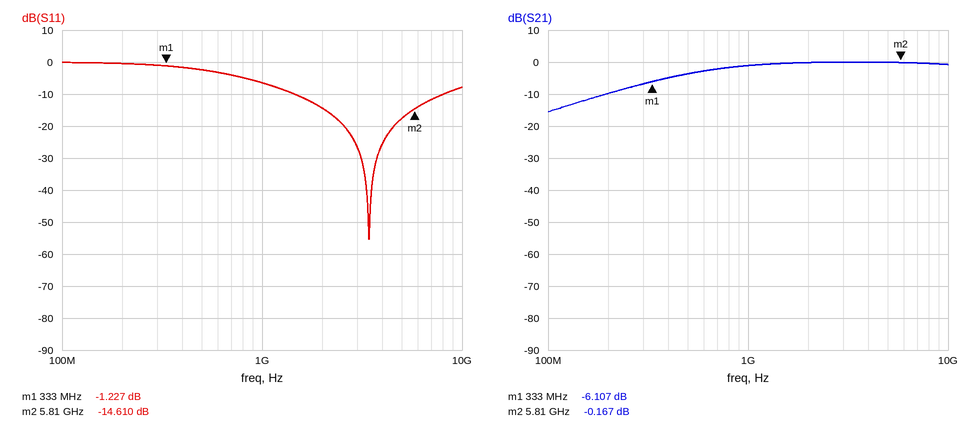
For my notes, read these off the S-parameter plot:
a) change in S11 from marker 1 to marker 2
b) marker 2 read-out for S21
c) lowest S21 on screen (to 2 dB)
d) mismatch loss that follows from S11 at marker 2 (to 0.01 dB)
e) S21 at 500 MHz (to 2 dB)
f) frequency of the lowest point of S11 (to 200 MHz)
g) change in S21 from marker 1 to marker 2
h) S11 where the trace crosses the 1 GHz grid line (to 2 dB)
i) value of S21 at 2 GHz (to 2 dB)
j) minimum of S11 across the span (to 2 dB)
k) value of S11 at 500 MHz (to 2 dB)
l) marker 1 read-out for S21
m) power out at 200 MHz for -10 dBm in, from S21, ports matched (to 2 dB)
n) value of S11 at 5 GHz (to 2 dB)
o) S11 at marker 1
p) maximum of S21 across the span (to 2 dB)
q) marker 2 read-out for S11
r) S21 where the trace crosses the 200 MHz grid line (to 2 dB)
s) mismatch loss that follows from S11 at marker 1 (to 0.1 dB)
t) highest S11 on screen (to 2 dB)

-13.383 dB
-0.167 dB
-16 dB
0.15 dB
-4 dB
3.4 GHz
5.940 dB
-6 dB
0 dB
-56 dB
-2 dB
-6.107 dB
-20 dBm
-18 dB
-1.227 dB
0 dB
-14.610 dB
-10 dB
6.1 dB
0 dB
